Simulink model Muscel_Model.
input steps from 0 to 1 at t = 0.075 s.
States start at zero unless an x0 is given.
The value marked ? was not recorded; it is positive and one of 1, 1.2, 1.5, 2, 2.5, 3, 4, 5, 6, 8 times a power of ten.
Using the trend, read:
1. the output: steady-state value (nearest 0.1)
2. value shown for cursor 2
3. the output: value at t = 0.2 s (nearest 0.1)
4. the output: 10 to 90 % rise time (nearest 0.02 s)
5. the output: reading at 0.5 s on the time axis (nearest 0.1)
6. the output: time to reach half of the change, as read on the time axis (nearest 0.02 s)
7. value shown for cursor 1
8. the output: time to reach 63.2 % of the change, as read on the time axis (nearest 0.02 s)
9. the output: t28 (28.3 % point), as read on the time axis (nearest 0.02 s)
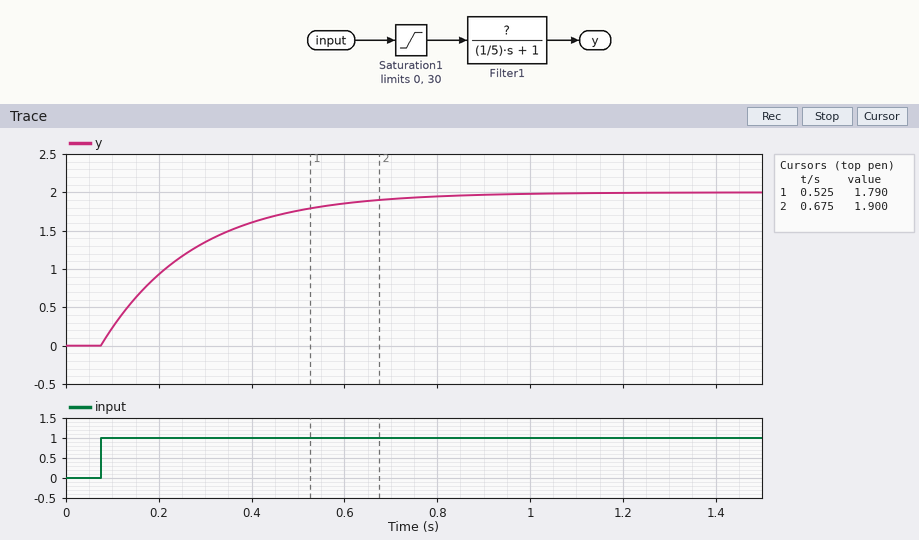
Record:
2.0
1.900
0.9
0.44 s
1.8
0.22 s
1.790
0.28 s
0.14 s
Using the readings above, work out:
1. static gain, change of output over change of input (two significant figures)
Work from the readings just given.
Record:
2.0
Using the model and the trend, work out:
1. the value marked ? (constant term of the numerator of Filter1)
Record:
2
